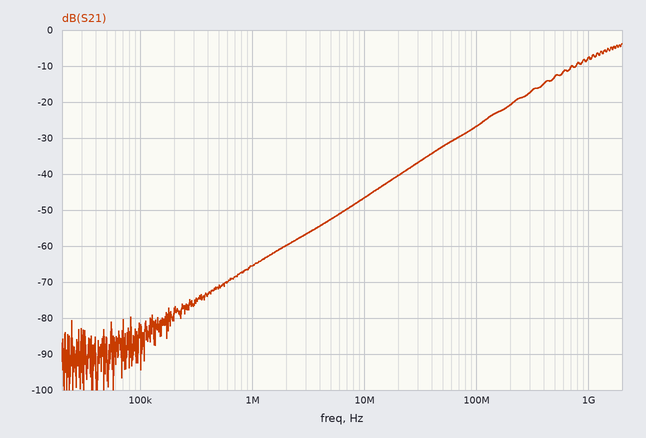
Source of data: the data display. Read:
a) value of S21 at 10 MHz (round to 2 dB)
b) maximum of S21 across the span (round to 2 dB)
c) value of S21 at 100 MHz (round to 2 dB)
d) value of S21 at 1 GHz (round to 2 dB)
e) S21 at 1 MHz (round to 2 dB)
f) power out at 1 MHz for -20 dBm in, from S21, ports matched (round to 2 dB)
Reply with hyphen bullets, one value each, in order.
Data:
- -46 dB
- -4 dB
- -26 dB
- -8 dB
- -66 dB
- -86 dBm
